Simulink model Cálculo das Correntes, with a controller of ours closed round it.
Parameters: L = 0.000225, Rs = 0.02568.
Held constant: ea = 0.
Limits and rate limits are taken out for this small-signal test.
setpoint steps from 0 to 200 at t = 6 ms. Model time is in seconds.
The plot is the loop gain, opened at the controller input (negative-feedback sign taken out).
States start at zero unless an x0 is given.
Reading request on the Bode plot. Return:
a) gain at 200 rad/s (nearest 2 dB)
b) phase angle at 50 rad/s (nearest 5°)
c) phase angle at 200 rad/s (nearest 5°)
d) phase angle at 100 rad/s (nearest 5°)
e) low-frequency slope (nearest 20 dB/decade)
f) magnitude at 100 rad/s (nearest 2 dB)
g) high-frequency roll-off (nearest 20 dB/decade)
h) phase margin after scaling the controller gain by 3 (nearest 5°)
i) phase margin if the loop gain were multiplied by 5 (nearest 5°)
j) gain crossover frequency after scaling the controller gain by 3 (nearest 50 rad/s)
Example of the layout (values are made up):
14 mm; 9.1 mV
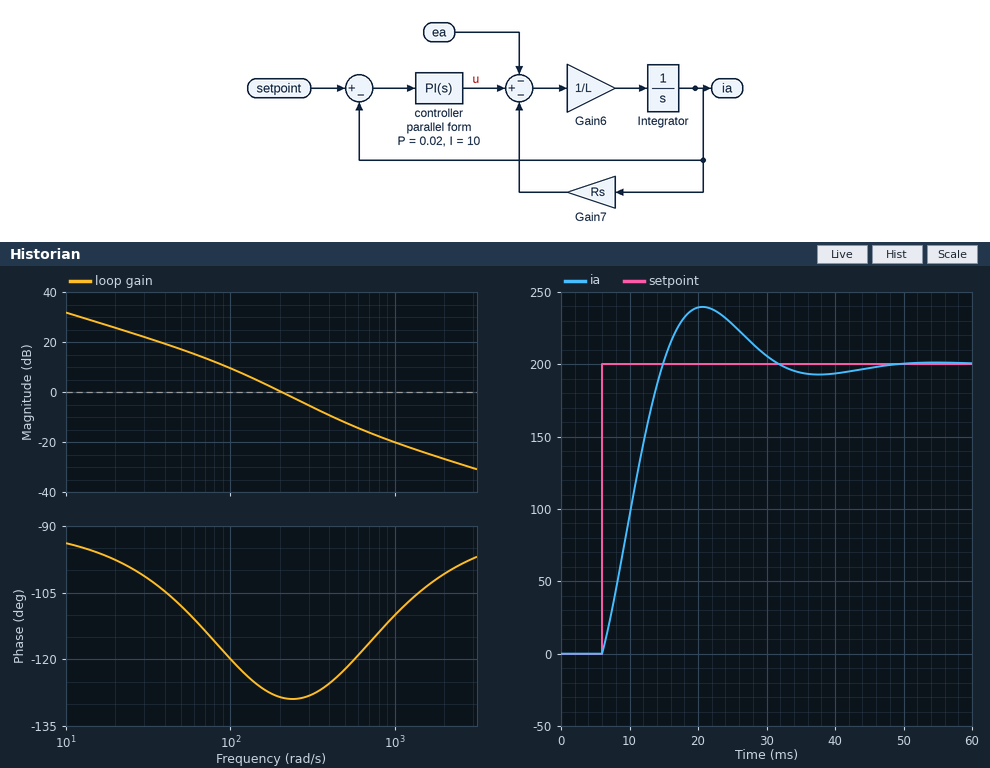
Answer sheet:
0 dB; -110°; -130°; -120°; -20 dB/decade; 10 dB; -20 dB/decade; 55°; 60°; 400 rad/s
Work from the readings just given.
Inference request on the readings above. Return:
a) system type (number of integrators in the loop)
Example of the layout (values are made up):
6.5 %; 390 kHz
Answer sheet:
1
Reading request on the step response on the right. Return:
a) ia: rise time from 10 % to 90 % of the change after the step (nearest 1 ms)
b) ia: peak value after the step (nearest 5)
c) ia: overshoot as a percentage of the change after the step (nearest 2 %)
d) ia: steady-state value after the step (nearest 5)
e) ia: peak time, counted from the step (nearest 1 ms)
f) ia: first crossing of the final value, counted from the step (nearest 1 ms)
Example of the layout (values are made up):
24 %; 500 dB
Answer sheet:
7 ms; 240; 20 %; 200; 15 ms; 9 ms
